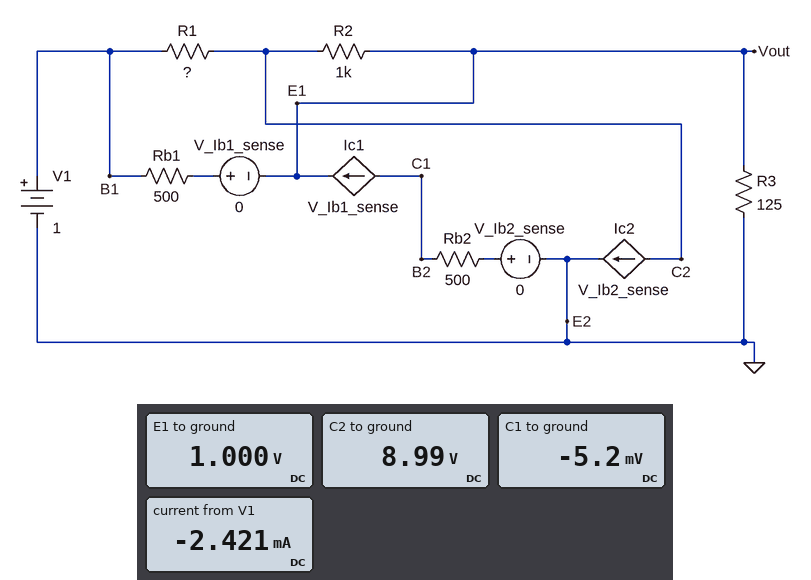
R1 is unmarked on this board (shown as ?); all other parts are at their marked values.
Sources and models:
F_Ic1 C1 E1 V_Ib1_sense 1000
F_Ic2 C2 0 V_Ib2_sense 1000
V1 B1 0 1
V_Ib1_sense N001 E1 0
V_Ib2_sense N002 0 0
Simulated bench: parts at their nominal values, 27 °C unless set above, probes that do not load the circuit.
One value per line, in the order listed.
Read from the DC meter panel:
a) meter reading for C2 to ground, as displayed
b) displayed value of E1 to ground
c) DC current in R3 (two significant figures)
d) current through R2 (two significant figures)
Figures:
8.99 V
1.000 V
8.0 mA
8.0 mA
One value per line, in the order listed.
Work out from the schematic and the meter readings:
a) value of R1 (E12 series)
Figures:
3.3 kΩ
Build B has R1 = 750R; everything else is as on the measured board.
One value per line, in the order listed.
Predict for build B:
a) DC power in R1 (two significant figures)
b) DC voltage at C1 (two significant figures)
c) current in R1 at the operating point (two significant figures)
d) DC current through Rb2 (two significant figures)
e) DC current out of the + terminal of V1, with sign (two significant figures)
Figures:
85 mW
-9.3 mV
11 mA
19 µA
-11 mA
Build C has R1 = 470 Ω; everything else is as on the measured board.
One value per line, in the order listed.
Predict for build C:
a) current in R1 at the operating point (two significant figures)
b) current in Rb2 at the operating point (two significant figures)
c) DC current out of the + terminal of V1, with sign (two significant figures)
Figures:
17 mA
25 µA
-17 mA
